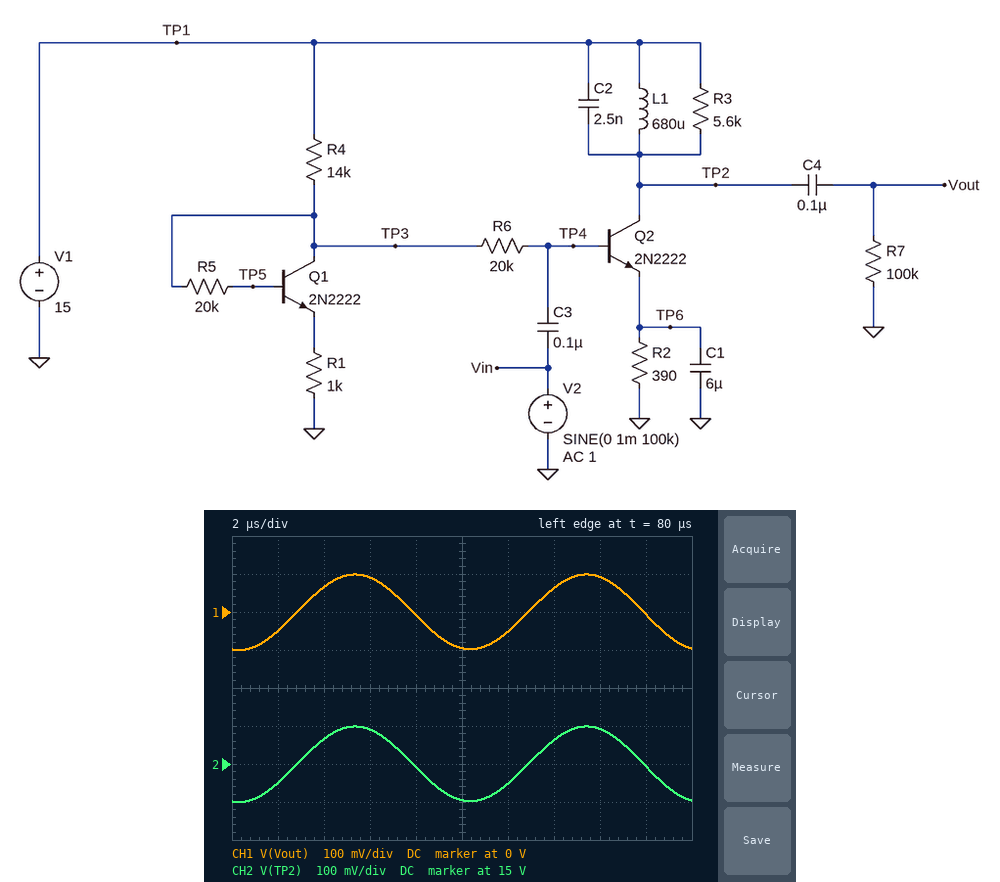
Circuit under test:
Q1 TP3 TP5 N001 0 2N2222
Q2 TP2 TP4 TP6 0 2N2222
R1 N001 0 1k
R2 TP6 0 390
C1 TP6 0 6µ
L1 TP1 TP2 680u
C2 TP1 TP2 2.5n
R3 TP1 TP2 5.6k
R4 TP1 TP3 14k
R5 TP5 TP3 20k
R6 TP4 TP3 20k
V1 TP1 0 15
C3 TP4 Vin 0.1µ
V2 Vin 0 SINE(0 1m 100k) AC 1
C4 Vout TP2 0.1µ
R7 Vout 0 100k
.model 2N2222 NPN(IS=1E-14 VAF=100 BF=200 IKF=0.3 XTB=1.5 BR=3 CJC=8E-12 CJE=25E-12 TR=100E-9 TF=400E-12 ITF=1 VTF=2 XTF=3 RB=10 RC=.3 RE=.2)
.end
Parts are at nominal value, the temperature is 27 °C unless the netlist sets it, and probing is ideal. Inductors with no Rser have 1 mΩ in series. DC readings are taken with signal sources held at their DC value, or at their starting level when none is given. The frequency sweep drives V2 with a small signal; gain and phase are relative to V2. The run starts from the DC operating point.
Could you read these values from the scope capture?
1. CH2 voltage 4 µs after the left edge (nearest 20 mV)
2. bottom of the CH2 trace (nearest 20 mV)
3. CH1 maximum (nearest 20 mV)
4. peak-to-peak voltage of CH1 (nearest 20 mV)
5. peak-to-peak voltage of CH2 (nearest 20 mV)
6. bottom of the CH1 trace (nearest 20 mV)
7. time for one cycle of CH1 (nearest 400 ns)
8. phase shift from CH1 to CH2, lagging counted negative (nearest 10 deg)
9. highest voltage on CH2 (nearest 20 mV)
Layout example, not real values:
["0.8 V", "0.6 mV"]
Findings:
["15.06 V", "14.90 V", "100 mV", "200 mV", "200 mV", "-100 mV", "10.0 µs", "0 deg", "15.10 V"]
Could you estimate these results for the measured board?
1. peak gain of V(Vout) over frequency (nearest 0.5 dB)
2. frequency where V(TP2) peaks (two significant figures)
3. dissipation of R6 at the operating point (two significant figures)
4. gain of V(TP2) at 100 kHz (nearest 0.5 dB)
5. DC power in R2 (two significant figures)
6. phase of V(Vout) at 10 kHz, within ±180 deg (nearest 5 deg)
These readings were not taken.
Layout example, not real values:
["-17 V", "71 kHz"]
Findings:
["51.5 dB", "120 kHz", "1.8 µW", "40.0 dB", "1.8 mW", "-75 deg"]
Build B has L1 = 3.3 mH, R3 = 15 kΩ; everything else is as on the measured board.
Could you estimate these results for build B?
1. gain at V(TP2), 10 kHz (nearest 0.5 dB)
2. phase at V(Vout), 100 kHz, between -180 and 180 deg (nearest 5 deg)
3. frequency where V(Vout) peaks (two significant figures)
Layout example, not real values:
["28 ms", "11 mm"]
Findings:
["24.5 dB", "95 deg", "55 kHz"]
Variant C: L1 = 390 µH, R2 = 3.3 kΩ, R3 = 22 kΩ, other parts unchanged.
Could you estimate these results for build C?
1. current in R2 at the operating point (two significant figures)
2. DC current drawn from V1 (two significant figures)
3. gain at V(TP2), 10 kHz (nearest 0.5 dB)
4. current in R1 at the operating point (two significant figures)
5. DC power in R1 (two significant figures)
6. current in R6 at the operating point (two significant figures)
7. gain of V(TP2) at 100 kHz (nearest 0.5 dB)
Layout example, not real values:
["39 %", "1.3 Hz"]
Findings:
["320 µA", "1.3 mA", "-10.5 dB", "950 µA", "900 µW", "1.4 µA", "13.5 dB"]
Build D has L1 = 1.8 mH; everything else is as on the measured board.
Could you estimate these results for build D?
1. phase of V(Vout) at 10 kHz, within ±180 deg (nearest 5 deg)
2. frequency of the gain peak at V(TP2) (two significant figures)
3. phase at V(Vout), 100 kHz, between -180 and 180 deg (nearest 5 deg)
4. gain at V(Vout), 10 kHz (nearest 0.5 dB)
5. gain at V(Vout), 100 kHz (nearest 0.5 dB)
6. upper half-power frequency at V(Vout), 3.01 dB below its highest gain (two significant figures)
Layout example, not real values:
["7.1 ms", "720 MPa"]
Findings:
["-75 deg", "75 kHz", "110 deg", "19.0 dB", "41.0 dB", "82 kHz"]
